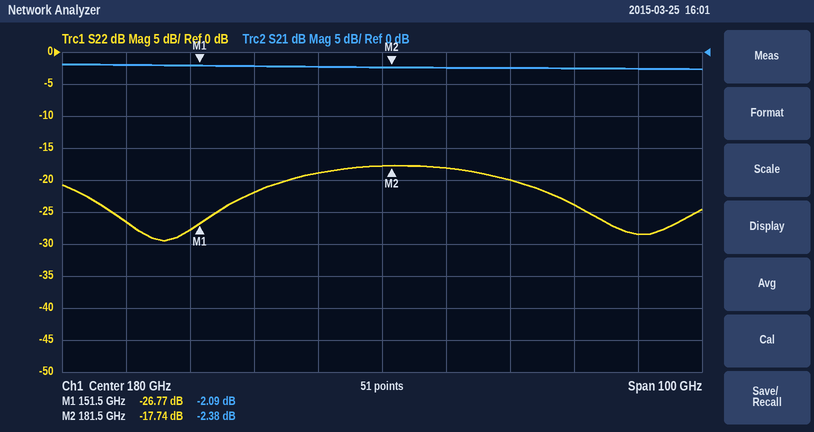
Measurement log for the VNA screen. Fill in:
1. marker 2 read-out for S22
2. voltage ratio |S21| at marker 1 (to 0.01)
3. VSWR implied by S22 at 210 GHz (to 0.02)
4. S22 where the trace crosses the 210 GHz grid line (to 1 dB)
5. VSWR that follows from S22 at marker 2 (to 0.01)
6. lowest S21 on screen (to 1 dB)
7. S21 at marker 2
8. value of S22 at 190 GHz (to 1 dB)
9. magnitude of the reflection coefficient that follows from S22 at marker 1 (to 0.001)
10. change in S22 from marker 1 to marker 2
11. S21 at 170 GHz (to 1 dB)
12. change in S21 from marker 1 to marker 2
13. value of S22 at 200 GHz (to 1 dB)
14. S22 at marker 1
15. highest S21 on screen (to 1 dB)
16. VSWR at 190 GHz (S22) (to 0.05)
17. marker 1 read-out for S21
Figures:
-17.74 dB
0.79
1.14
-24 dB
1.30
-3 dB
-2.38 dB
-18 dB
0.046
9.03 dB
-2 dB
-0.29 dB
-20 dB
-26.77 dB
-2 dB
1.30
-2.09 dB
